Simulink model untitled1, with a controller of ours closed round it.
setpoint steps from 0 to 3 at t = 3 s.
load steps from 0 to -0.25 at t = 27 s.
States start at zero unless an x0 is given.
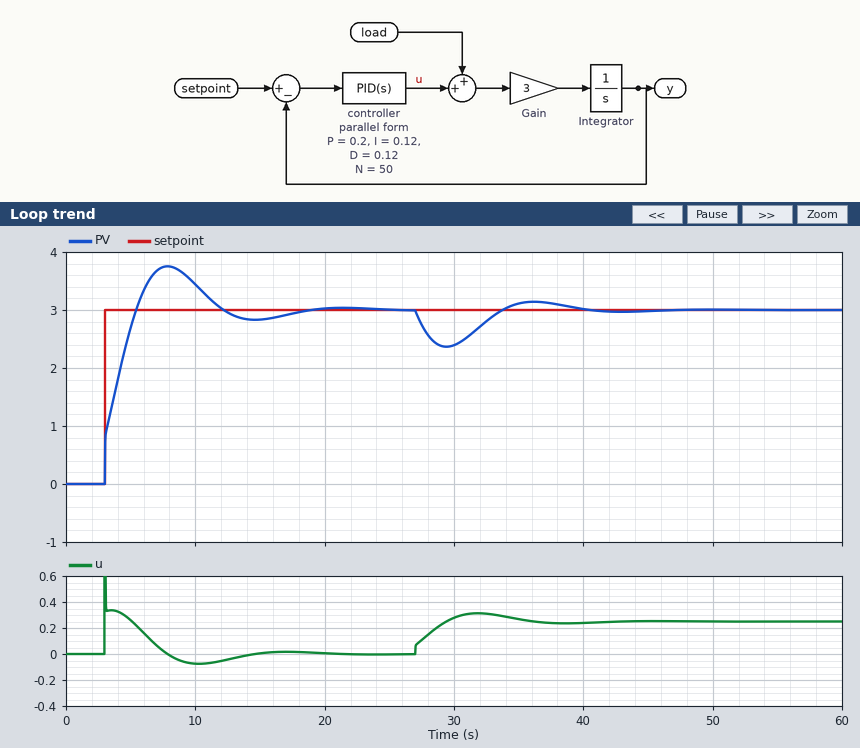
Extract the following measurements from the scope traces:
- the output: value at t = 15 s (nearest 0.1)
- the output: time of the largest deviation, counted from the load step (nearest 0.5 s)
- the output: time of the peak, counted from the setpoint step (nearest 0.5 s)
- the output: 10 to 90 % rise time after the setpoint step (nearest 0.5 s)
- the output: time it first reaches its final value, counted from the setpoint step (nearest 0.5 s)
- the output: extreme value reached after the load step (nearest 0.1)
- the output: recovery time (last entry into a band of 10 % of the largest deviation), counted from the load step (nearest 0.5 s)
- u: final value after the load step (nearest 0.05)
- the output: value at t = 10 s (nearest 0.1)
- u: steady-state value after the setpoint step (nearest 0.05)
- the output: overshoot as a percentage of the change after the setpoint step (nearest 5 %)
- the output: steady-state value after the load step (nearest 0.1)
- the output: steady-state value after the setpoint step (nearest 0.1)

2.8
2.5 s
5.0 s
2.0 s
2.5 s
2.4
12.0 s
0.25
3.4
0.00
25 %
3.0
3.0
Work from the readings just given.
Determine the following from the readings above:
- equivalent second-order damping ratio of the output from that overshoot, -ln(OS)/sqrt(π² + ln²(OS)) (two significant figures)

0.40
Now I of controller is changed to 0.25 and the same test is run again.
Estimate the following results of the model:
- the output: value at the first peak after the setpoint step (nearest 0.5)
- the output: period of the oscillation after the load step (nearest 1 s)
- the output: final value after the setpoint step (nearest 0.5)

4.0
9 s
3.0
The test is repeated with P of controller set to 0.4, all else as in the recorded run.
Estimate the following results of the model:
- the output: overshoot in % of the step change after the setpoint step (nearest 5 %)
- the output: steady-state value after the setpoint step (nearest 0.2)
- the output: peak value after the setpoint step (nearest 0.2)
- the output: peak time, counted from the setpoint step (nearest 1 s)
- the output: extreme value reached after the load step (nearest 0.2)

10 %
3.0
3.4
4 s
2.6
